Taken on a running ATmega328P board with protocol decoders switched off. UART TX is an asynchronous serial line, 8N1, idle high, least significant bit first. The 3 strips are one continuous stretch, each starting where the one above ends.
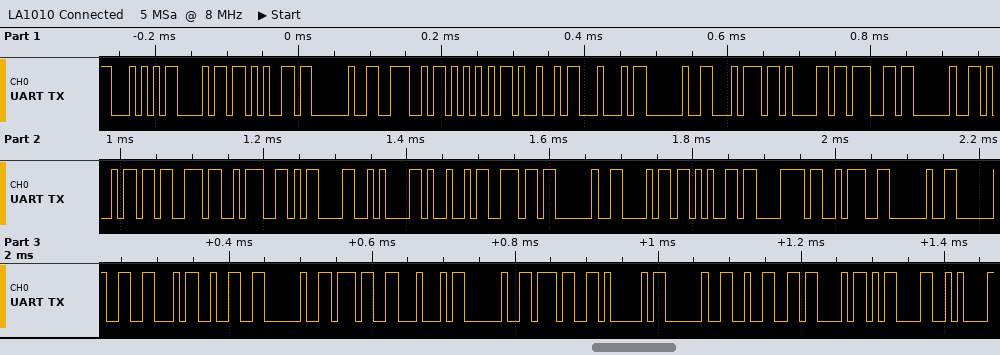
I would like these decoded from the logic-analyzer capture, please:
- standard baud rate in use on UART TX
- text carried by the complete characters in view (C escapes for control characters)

115200 baud
"The NUID tag is:\r\nIn hex:  F2 7D 7A 2C\r\n"
